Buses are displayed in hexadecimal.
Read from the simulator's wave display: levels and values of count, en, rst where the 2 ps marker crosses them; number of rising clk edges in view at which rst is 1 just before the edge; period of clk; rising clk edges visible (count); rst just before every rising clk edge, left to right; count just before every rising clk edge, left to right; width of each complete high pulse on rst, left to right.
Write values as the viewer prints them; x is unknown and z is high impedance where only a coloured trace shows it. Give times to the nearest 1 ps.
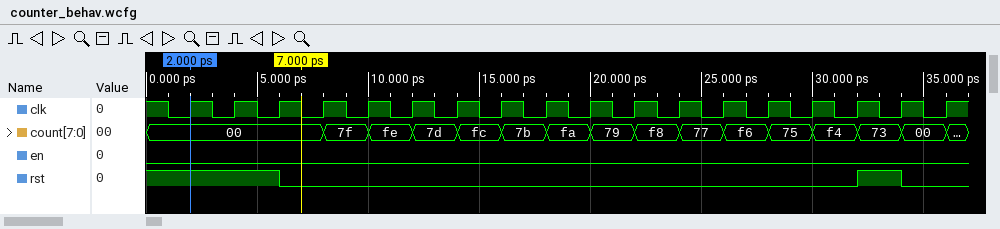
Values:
count=00, en=0, rst=1
4
2 ps
18
1 1 1 0 0 0 0 0 0 0 0 0 0 0 0 0 1 0
00, 00, 00, 00, 7f, fe, 7d, fc, 7b, fa, 79, f8, 77, f6, 75, f4, 73, 00
2 ps
